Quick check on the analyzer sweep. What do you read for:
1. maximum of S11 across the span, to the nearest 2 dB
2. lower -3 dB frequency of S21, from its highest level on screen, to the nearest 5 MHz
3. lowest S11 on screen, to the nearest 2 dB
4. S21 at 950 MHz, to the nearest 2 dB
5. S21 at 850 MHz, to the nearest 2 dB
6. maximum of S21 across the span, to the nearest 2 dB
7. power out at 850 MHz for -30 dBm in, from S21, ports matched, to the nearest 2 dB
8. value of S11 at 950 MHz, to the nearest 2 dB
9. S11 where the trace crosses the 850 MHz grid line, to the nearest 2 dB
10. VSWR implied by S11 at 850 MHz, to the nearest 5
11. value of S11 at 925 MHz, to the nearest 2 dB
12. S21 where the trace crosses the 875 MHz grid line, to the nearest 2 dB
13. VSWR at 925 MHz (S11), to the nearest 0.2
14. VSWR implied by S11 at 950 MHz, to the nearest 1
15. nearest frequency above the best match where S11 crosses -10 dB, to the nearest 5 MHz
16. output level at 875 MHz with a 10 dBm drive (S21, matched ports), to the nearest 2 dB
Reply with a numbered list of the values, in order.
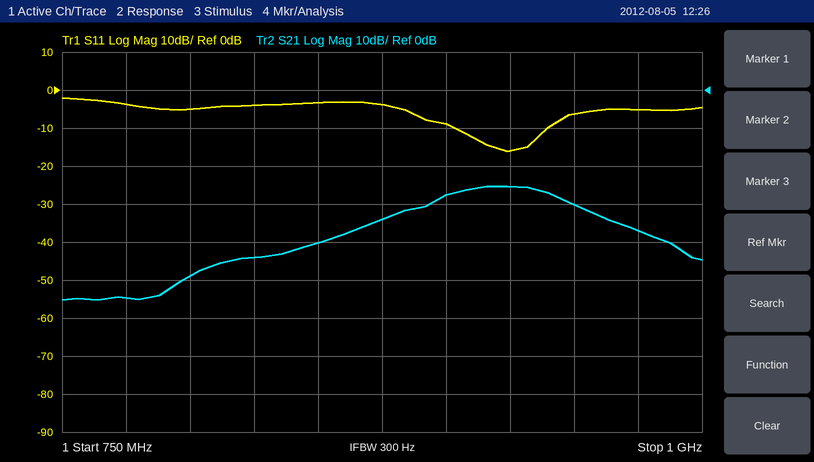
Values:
1. -2 dB
2. 900 MHz
3. -16 dB
4. -30 dB
5. -40 dB
6. -26 dB
7. -70 dBm
8. -6 dB
9. -4 dB
10. 5
11. -16 dB
12. -34 dB
13. 1.4
14. 3
15. 940 MHz
16. -24 dBm
